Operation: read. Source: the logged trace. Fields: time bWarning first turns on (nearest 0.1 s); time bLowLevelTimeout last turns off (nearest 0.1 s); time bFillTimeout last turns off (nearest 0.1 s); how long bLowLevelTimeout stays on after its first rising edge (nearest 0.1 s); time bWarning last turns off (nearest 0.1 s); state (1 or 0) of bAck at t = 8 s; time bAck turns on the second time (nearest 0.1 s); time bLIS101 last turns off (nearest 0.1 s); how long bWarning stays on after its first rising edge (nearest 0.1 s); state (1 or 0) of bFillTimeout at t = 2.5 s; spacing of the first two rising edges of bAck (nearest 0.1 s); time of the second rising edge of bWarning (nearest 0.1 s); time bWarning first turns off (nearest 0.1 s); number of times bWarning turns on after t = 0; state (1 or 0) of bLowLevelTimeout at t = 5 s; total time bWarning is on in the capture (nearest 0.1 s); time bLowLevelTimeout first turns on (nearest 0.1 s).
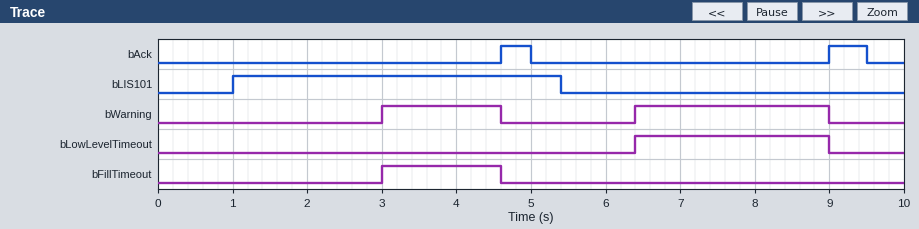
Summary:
3.0 s
9.0 s
4.6 s
2.6 s
9.0 s
0
9.0 s
5.4 s
1.6 s
0
4.4 s
6.4 s
4.6 s
2
0
4.2 s
6.4 s
